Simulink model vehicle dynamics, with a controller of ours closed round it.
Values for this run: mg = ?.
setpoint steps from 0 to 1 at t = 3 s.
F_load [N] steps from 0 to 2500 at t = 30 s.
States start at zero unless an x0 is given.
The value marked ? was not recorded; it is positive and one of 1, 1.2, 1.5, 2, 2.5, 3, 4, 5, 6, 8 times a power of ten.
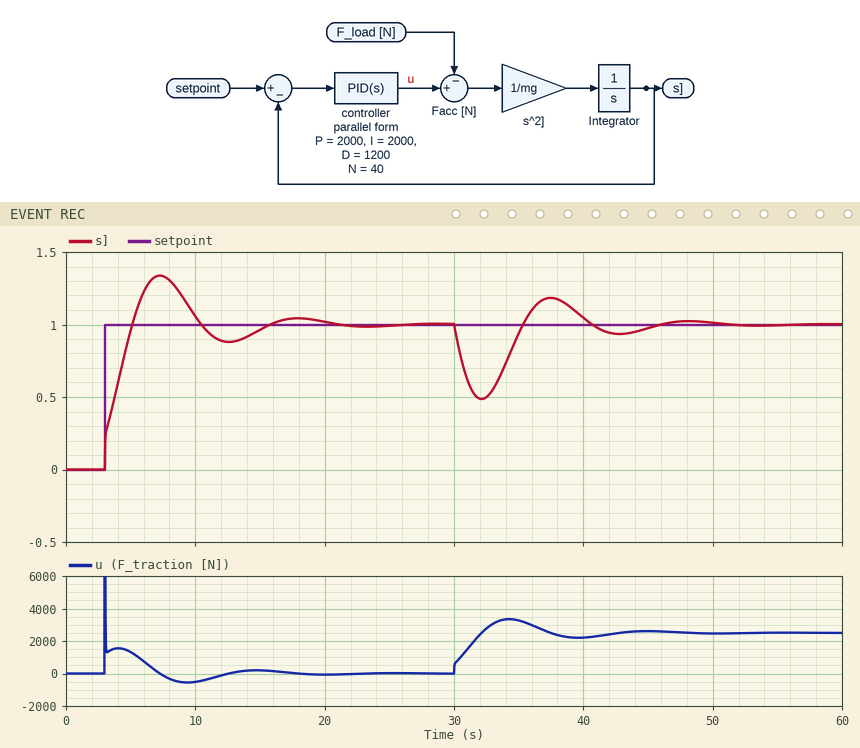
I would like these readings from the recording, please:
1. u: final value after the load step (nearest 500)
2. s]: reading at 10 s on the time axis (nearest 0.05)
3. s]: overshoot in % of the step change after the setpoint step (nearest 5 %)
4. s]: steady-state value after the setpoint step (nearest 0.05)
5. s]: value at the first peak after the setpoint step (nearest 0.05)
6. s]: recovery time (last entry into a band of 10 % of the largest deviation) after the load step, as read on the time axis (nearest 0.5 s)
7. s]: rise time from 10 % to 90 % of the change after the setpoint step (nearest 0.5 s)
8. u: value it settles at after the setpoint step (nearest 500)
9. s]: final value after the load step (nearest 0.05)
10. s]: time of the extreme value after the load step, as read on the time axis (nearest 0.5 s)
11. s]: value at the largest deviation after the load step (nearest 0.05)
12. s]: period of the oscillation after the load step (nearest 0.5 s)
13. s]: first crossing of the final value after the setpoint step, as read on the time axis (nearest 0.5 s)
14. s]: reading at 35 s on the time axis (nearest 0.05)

2500
1.05
35 %
1.00
1.35
44.0 s
2.0 s
0
1.00
32.0 s
0.50
10.5 s
5.0 s
0.95
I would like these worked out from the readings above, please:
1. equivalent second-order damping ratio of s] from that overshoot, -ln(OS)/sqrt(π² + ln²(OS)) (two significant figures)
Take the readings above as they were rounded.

0.32
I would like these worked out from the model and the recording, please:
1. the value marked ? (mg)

4000
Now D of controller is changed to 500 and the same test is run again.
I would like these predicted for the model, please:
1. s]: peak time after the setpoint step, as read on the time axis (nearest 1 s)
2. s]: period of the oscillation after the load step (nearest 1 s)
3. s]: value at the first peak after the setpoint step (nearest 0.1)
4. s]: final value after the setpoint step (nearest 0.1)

7 s
10 s
1.4
1.0
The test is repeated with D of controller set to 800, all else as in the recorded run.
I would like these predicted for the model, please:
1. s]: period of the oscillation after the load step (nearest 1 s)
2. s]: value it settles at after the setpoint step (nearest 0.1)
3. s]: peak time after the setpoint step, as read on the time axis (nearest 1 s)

10 s
1.0
7 s
